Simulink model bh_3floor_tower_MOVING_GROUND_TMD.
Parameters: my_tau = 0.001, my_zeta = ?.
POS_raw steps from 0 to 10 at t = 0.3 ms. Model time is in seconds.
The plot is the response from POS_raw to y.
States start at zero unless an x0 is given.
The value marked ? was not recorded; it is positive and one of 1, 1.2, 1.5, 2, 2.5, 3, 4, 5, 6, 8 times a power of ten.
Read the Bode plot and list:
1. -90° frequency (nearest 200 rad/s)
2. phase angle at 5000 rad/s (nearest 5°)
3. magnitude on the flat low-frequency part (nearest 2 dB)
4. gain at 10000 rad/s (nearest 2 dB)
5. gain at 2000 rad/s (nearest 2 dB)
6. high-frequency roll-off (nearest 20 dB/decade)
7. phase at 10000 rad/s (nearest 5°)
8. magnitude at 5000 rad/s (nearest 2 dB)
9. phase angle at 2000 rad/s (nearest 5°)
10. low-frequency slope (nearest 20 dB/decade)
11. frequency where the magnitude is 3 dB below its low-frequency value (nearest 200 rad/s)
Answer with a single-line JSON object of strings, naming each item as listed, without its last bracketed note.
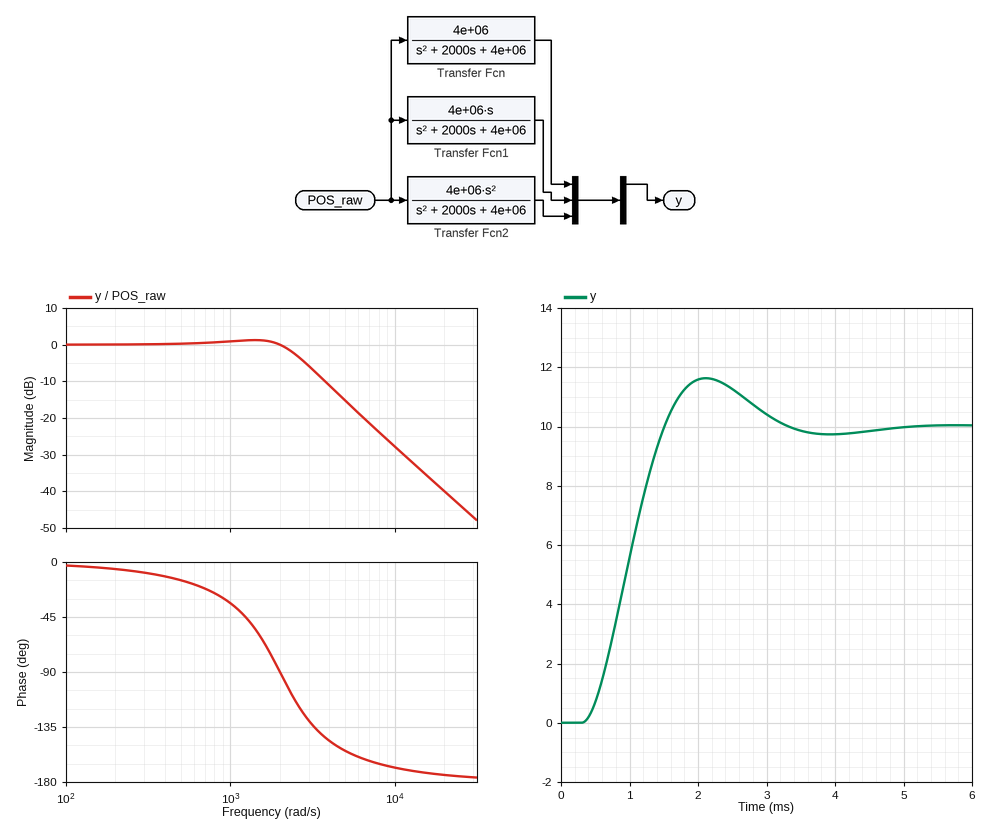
{"-90° frequency": "2000 rad/s", "phase angle at 5000 rad/s": "-155°", "magnitude on the flat low-frequency part": "0 dB", "gain at 10000 rad/s": "-28 dB", "gain at 2000 rad/s": "0 dB", "high-frequency roll-off": "-40 dB/decade", "phase at 10000 rad/s": "-170°", "magnitude at 5000 rad/s": "-16 dB", "phase angle at 2000 rad/s": "-90°", "low-frequency slope": "0 dB/decade", "frequency where the magnitude is 3 dB below its low-frequency value": "2600 rad/s"}
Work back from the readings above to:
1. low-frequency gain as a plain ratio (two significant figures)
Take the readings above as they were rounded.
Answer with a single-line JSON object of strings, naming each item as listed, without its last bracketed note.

{"low-frequency gain as a plain ratio": "1.0"}
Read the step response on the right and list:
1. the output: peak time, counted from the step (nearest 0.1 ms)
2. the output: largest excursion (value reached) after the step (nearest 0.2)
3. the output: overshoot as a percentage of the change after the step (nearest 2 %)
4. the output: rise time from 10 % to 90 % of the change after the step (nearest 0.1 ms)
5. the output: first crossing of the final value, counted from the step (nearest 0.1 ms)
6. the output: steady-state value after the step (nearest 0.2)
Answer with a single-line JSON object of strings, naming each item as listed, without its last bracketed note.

{"the output: peak time, counted from the step": "1.8 ms", "the output: largest excursion (value reached) after the step": "11.6", "the output: overshoot as a percentage of the change after the step": "16 %", "the output: rise time from 10 % to 90 % of the change after the step": "0.8 ms", "the output: first crossing of the final value, counted from the step": "1.2 ms", "the output: steady-state value after the step": "10.0"}
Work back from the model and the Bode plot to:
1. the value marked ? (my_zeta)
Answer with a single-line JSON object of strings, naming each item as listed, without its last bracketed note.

{"the value marked ?": "0.5"}
